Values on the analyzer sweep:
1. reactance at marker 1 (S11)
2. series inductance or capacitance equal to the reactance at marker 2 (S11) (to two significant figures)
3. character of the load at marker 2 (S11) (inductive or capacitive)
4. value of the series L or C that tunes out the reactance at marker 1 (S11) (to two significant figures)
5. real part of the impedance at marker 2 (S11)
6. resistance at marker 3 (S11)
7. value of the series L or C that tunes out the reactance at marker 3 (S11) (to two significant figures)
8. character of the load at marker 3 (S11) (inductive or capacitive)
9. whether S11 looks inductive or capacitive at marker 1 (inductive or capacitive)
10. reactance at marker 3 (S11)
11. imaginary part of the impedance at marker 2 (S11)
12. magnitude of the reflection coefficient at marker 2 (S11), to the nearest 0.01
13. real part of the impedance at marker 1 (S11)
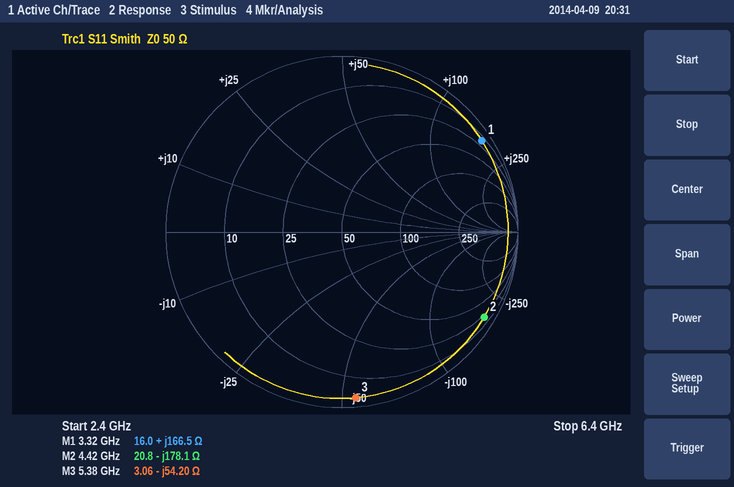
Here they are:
+166.5 Ω
200 fF
capacitive
290 fF
20.8 Ω
3.06 Ω
1.6 nH
capacitive
inductive
-54.20 Ω
-178.1 Ω
0.94
16.0 Ω
